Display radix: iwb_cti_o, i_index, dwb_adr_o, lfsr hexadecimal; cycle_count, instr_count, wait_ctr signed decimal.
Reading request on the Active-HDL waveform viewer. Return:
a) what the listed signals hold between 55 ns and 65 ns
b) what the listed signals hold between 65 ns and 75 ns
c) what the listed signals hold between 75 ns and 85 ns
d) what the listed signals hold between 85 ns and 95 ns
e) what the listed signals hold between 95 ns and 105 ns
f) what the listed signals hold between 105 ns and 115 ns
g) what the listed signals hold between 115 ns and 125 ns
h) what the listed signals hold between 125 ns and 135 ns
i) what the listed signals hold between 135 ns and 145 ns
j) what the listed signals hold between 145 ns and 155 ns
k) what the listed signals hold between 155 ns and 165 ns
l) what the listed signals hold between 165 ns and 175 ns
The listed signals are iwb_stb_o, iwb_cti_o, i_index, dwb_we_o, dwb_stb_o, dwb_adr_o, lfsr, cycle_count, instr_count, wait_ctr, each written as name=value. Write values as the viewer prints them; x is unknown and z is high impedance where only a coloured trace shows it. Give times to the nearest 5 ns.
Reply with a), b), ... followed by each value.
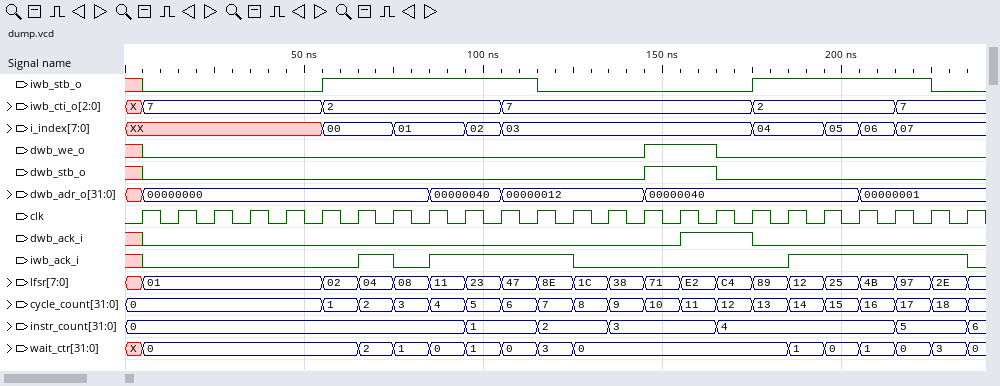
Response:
a) iwb_stb_o=1, iwb_cti_o=2, i_index=00, dwb_we_o=0, dwb_stb_o=0, dwb_adr_o=00000000, lfsr=02, cycle_count=1, instr_count=0, wait_ctr=0
b) iwb_stb_o=1, iwb_cti_o=2, i_index=00, dwb_we_o=0, dwb_stb_o=0, dwb_adr_o=00000000, lfsr=04, cycle_count=2, instr_count=0, wait_ctr=2
c) iwb_stb_o=1, iwb_cti_o=2, i_index=01, dwb_we_o=0, dwb_stb_o=0, dwb_adr_o=00000000, lfsr=08, cycle_count=3, instr_count=0, wait_ctr=1
d) iwb_stb_o=1, iwb_cti_o=2, i_index=01, dwb_we_o=0, dwb_stb_o=0, dwb_adr_o=00000040, lfsr=11, cycle_count=4, instr_count=0, wait_ctr=0
e) iwb_stb_o=1, iwb_cti_o=2, i_index=02, dwb_we_o=0, dwb_stb_o=0, dwb_adr_o=00000040, lfsr=23, cycle_count=5, instr_count=1, wait_ctr=1
f) iwb_stb_o=1, iwb_cti_o=7, i_index=03, dwb_we_o=0, dwb_stb_o=0, dwb_adr_o=00000012, lfsr=47, cycle_count=6, instr_count=1, wait_ctr=0
g) iwb_stb_o=0, iwb_cti_o=7, i_index=03, dwb_we_o=0, dwb_stb_o=0, dwb_adr_o=00000012, lfsr=8E, cycle_count=7, instr_count=2, wait_ctr=3
h) iwb_stb_o=0, iwb_cti_o=7, i_index=03, dwb_we_o=0, dwb_stb_o=0, dwb_adr_o=00000012, lfsr=1C, cycle_count=8, instr_count=2, wait_ctr=0
i) iwb_stb_o=0, iwb_cti_o=7, i_index=03, dwb_we_o=0, dwb_stb_o=0, dwb_adr_o=00000012, lfsr=38, cycle_count=9, instr_count=3, wait_ctr=0
j) iwb_stb_o=0, iwb_cti_o=7, i_index=03, dwb_we_o=1, dwb_stb_o=1, dwb_adr_o=00000040, lfsr=71, cycle_count=10, instr_count=3, wait_ctr=0
k) iwb_stb_o=0, iwb_cti_o=7, i_index=03, dwb_we_o=1, dwb_stb_o=1, dwb_adr_o=00000040, lfsr=E2, cycle_count=11, instr_count=3, wait_ctr=0
l) iwb_stb_o=0, iwb_cti_o=7, i_index=03, dwb_we_o=0, dwb_stb_o=0, dwb_adr_o=00000040, lfsr=C4, cycle_count=12, instr_count=4, wait_ctr=0
